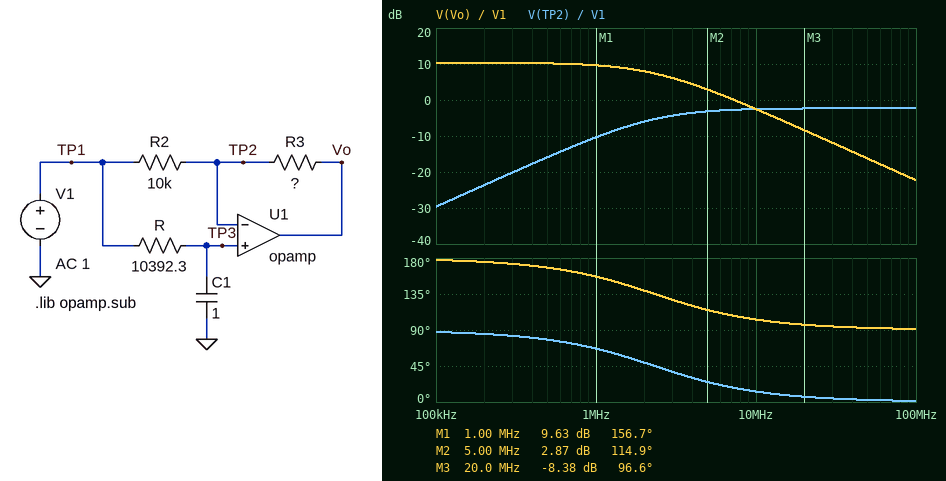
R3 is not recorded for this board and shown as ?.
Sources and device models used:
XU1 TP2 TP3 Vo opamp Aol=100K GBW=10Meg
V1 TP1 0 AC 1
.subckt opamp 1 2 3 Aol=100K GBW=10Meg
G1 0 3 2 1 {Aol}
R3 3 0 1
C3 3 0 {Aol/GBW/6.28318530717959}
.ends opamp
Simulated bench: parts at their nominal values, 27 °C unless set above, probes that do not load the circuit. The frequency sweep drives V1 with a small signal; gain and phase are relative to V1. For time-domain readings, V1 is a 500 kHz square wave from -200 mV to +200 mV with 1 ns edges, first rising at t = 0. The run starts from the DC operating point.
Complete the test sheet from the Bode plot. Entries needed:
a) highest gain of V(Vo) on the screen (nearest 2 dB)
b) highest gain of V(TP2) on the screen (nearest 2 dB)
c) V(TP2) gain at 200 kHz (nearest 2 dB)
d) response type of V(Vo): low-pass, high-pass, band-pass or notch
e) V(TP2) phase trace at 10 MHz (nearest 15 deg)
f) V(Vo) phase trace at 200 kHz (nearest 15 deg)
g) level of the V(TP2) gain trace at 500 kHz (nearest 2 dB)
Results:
10 dB
-2 dB
-24 dB
low-pass
15 deg
180 deg
-16 dB
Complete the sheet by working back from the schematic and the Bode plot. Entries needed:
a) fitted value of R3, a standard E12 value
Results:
33 kΩ
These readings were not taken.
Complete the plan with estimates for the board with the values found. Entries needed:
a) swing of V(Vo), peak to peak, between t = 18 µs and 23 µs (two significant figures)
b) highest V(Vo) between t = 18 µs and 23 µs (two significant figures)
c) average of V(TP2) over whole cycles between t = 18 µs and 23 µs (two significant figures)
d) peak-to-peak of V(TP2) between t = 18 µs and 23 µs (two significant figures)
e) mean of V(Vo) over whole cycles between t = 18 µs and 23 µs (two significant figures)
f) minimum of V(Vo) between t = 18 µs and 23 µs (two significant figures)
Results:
1.3 V
-200 mV
-200 mV
610 mV
-860 mV
-1.5 V
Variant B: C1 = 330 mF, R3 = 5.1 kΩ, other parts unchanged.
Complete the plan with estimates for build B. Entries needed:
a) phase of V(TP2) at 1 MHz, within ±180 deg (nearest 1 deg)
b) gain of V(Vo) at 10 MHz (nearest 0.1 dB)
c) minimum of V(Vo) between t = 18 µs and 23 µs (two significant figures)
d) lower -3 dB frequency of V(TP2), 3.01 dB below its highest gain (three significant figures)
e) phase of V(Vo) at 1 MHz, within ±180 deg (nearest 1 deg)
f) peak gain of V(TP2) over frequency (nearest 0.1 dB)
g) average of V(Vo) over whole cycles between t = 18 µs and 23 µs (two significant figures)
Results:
81 deg
-11.0 dB
-400 mV
6.62 MHz
171 deg
-9.4 dB
-300 mV
